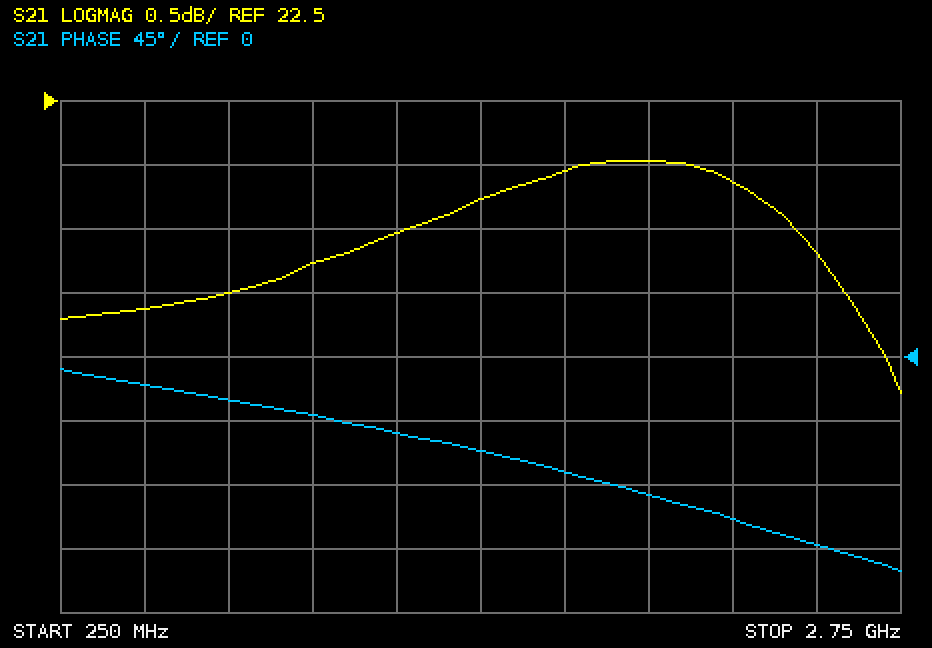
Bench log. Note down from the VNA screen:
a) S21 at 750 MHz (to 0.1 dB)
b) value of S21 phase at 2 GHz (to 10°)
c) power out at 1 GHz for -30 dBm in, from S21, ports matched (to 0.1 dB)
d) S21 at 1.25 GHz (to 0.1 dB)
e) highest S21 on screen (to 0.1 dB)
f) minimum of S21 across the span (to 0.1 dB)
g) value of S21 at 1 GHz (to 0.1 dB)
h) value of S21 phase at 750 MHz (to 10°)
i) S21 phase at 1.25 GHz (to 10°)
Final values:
21.0 dB
-100°
-8.8 dBm
21.5 dB
22.0 dB
20.2 dB
21.2 dB
-30°
-50°
